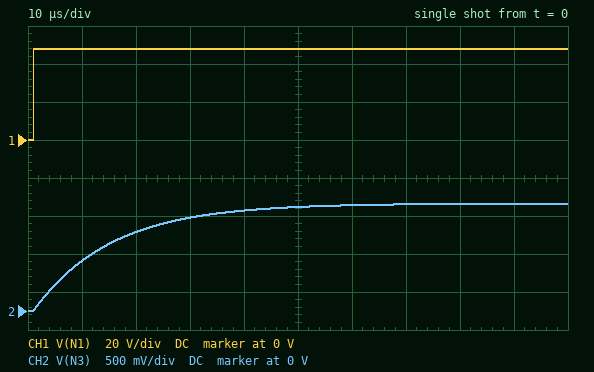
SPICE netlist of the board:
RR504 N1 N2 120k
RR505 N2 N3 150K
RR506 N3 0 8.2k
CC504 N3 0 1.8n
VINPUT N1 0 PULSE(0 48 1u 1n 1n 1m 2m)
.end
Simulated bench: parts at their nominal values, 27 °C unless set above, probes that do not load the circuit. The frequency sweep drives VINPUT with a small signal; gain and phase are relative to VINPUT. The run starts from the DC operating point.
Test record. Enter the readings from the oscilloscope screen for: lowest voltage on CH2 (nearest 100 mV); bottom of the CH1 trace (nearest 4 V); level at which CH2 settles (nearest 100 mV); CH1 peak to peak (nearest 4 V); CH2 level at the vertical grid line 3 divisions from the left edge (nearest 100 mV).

0 V
0 V
1.4 V
48 V
1.2 V
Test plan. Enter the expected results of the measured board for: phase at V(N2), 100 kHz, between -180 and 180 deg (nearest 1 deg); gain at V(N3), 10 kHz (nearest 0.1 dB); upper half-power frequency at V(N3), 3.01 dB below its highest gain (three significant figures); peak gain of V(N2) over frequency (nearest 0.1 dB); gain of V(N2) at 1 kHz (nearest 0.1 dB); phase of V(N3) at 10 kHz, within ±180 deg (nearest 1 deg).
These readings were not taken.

0 deg
-33.2 dB
11.1 kHz
-4.9 dB
-4.9 dB
-42 deg
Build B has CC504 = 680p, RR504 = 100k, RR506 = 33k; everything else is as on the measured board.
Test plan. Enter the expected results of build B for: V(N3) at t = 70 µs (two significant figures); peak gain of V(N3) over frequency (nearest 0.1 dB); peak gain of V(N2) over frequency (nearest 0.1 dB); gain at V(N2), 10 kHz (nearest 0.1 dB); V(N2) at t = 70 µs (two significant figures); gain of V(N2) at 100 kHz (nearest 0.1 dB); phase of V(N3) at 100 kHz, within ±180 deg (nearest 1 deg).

5.4 V
-18.7 dB
-3.8 dB
-4.2 dB
31 V
-4.4 dB
-85 deg
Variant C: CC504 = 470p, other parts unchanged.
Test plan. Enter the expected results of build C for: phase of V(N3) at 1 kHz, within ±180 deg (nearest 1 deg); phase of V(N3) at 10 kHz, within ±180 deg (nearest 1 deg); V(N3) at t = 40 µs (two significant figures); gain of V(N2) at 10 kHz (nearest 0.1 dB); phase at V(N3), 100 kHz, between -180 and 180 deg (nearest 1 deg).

-1 deg
-13 deg
1.4 V
-4.9 dB
-67 deg
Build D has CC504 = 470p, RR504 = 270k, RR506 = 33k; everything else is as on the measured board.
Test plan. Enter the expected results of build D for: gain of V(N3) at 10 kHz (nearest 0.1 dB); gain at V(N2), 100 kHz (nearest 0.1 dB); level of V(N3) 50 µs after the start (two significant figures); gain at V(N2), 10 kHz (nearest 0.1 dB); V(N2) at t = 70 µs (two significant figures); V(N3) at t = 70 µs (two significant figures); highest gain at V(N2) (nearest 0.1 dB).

-25.3 dB
-8.9 dB
3.4 V
-8.3 dB
19 V
3.5 V
-7.9 dB
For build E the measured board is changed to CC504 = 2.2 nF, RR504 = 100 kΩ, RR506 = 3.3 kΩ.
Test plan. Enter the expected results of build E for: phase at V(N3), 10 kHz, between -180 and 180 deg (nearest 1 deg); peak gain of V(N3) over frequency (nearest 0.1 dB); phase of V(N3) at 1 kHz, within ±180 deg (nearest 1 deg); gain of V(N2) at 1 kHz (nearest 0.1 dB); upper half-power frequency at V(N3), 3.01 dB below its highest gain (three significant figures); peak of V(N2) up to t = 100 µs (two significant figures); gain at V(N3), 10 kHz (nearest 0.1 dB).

-24 deg
-37.7 dB
-3 deg
-4.4 dB
22.2 kHz
29 V
-38.5 dB
